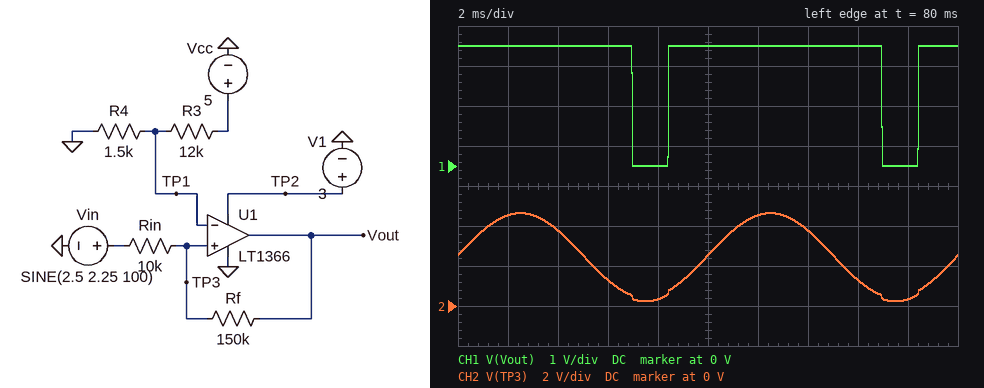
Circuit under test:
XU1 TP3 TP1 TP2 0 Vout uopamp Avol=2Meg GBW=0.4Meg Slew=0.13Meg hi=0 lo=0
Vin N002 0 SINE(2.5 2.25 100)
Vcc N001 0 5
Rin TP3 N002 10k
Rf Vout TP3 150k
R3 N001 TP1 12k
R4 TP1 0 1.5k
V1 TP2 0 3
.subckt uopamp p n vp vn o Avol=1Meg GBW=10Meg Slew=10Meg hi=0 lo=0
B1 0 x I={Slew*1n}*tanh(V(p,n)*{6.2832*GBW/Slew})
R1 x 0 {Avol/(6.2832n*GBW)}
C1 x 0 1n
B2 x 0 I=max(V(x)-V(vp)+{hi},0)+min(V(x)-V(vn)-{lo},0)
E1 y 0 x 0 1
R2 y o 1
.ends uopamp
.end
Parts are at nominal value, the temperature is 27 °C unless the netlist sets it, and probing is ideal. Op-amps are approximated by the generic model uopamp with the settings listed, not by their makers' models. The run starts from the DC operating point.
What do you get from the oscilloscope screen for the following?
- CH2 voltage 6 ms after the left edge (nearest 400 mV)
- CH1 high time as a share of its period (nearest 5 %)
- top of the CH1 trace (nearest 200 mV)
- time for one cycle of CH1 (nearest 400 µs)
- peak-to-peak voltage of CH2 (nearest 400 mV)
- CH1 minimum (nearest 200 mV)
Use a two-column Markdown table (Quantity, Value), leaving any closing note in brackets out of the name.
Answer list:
| Quantity | Value |
|---|---|
| CH2 voltage 6 ms after the left edge | 1.2 V |
| CH1 high time as a share of its period | 85 % |
| top of the CH1 trace | 3.0 V |
| time for one cycle of CH1 | 10.0 ms |
| peak-to-peak voltage of CH2 | 4.4 V |
| CH1 minimum | 0 V |
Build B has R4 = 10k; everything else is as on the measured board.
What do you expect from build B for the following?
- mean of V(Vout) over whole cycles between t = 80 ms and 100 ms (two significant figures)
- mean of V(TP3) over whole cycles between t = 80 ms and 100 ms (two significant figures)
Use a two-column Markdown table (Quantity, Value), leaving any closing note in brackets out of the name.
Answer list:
| Quantity | Value |
|---|---|
| mean of V(Vout) over whole cycles between t = 80 ms and 100 ms | 1.6 V |
| mean of V(TP3) over whole cycles between t = 80 ms and 100 ms | 2.4 V |
